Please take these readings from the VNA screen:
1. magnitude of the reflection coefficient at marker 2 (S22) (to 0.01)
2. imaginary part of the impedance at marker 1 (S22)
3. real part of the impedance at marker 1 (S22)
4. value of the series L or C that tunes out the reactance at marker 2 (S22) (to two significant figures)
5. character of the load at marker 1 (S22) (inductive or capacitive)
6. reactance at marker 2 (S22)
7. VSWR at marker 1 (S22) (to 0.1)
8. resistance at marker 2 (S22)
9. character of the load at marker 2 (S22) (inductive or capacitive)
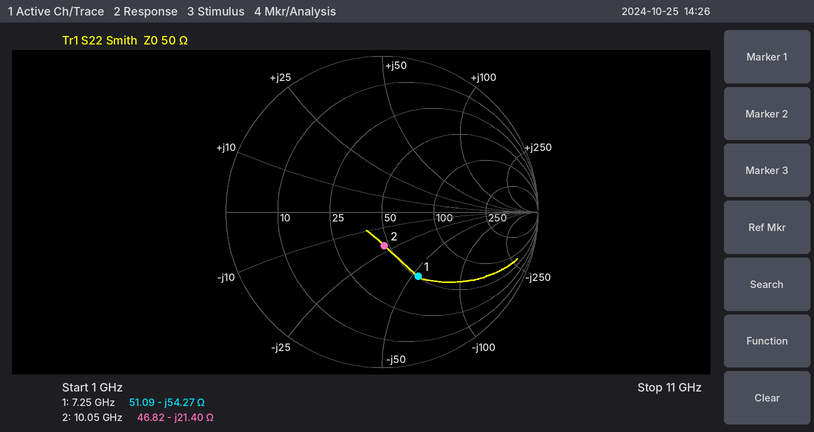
0.22
-54.27 Ω
51.09 Ω
340 pH
capacitive
-21.40 Ω
2.8
46.82 Ω
capacitive
